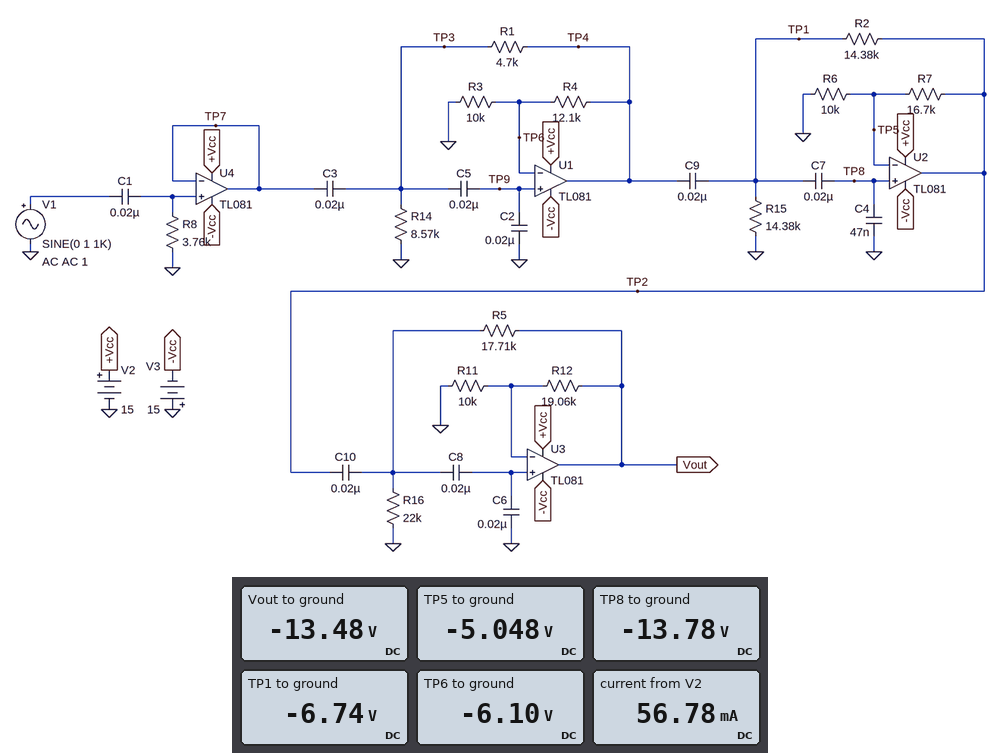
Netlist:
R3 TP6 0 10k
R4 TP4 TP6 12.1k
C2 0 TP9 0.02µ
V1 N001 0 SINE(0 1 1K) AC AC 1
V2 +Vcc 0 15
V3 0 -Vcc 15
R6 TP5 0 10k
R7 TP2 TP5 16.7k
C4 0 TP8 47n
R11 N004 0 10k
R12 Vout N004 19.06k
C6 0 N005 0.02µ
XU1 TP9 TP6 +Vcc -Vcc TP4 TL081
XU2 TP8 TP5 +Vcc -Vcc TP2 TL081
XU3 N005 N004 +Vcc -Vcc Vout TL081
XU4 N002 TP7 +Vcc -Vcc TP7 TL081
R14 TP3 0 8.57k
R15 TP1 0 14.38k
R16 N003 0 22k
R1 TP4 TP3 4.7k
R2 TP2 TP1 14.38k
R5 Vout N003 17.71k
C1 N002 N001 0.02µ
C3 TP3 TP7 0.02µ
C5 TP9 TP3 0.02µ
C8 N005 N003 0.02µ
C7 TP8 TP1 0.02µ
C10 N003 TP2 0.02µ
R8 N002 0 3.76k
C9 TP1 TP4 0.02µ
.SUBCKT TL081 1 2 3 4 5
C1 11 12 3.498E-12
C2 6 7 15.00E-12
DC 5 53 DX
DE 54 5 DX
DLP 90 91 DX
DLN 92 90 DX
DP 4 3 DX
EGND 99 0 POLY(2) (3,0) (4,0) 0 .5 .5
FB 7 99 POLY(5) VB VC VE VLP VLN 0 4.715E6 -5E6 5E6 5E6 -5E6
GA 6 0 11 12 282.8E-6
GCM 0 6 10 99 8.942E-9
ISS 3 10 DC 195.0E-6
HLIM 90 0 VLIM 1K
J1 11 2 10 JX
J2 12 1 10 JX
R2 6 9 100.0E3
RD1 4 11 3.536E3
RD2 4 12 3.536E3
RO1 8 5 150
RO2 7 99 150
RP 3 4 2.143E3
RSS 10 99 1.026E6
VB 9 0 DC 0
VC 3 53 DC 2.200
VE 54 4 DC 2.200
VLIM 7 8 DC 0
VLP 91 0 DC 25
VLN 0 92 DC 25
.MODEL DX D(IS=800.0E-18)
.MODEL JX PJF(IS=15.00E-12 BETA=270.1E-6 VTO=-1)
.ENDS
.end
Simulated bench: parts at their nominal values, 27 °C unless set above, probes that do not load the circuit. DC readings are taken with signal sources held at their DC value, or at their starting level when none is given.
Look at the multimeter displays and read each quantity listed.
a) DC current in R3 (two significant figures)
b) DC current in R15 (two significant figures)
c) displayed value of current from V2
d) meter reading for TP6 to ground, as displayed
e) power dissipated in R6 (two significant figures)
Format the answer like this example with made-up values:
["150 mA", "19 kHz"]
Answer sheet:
["610 µA", "470 µA", "56.78 mA", "-6.10 V", "2.5 mW"]
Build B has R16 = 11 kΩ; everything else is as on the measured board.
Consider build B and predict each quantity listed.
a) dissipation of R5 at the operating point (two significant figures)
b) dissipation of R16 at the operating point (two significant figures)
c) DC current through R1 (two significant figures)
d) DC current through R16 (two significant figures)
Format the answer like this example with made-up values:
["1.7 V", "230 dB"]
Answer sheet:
["3.9 mW", "2.4 mW", "1.0 mA", "470 µA"]
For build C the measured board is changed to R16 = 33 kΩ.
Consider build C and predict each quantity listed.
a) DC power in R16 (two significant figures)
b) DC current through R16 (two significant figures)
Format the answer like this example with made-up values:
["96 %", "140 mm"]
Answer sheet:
["2.3 mW", "270 µA"]
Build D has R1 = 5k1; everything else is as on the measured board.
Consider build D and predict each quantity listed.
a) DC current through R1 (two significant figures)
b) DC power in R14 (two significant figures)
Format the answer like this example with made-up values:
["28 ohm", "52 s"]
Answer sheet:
["990 µA", "8.3 mW"]
